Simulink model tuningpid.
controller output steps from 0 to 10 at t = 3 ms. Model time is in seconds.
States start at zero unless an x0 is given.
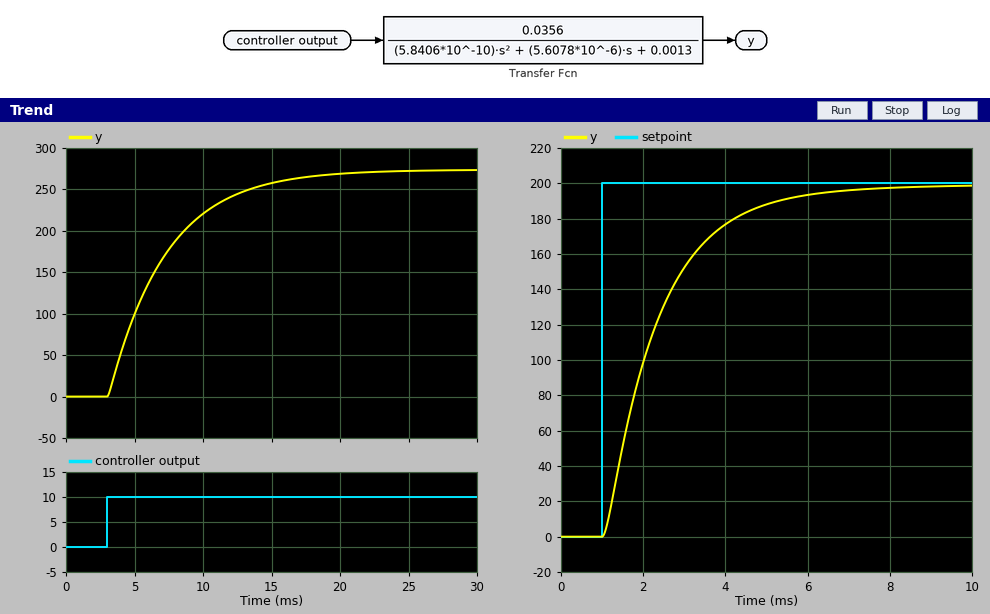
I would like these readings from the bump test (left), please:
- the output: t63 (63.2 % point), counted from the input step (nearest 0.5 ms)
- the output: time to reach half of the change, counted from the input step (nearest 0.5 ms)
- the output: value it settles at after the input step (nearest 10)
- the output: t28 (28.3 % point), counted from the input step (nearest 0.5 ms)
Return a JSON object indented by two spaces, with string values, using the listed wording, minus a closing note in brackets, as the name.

{
  "the output: t63 (63.2 % point), counted from the input step": "4.5 ms",
  "the output: time to reach half of the change, counted from the input step": "3.0 ms",
  "the output: value it settles at after the input step": "270",
  "the output: t28 (28.3 % point), counted from the input step": "1.5 ms"
}
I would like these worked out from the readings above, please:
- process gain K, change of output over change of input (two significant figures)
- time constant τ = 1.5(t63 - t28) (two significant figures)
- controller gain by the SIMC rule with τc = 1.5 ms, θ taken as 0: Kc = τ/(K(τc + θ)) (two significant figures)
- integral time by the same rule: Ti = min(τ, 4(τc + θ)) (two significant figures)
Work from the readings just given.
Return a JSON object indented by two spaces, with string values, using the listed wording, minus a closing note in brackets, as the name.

{
  "process gain K, change of output over change of input": "27",
  "time constant τ = 1.5(t63 - t28)": "4.5 ms",
  "controller gain by the SIMC rule with τc = 1.5 ms, θ taken as 0: Kc = τ/(K(τc + θ))": "0.11",
  "integral time by the same rule: Ti = min(τ, 4(τc + θ))": "4.5 ms"
}
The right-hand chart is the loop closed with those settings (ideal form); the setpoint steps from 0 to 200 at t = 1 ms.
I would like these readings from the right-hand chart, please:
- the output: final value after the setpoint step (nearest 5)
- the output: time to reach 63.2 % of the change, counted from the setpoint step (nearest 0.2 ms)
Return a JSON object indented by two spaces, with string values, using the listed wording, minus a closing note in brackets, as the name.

{
  "the output: final value after the setpoint step": "200",
  "the output: time to reach 63.2 % of the change, counted from the setpoint step": "1.4 ms"
}
